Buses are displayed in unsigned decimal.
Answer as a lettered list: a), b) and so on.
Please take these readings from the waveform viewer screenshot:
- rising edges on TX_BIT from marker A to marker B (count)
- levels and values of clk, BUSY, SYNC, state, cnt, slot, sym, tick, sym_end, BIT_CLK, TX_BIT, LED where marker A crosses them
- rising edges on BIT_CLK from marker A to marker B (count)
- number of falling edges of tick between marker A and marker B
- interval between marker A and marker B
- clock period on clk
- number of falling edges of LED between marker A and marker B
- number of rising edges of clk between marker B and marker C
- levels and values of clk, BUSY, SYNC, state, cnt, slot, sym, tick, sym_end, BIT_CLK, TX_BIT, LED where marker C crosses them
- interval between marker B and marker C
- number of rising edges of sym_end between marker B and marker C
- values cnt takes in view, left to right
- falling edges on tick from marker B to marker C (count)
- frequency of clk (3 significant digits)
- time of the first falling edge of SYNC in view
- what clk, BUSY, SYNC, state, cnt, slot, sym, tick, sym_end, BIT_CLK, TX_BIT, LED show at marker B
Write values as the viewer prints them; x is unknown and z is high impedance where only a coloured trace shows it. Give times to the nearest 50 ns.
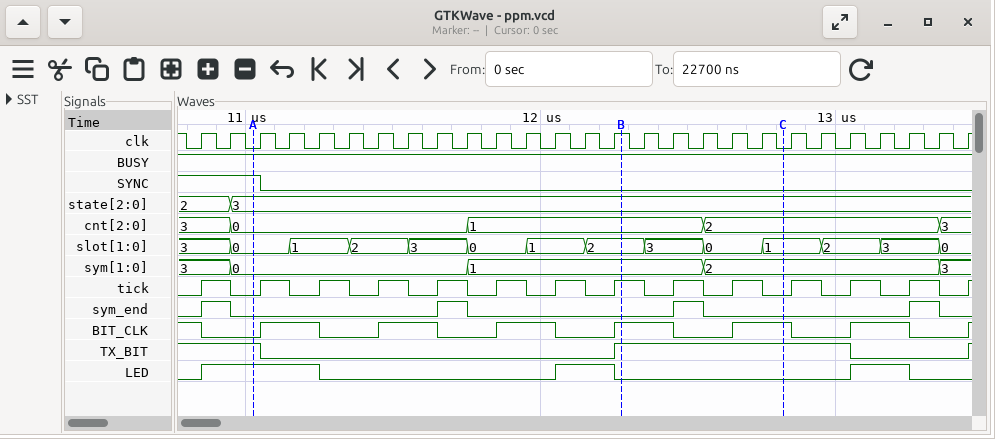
a) 1
b) clk=0, BUSY=1, SYNC=1, state=3, cnt=0, slot=0, sym=0, tick=0, sym_end=0, BIT_CLK=0, TX_BIT=1, LED=1
c) 4
d) 6
e) 1250 ns
f) 100 ns
g) 2
h) 5
i) clk=0, BUSY=1, SYNC=0, state=3, cnt=2, slot=1, sym=2, tick=0, sym_end=0, BIT_CLK=1, TX_BIT=1, LED=0
j) 550 ns
k) 1
l) 3, 0, 1, 2, 3
m) 3
n) 10.0 MHz
o) 11050 ns
p) clk=1, BUSY=1, SYNC=0, state=3, cnt=1, slot=2, sym=1, tick=1, sym_end=0, BIT_CLK=1, TX_BIT=1, LED=0
